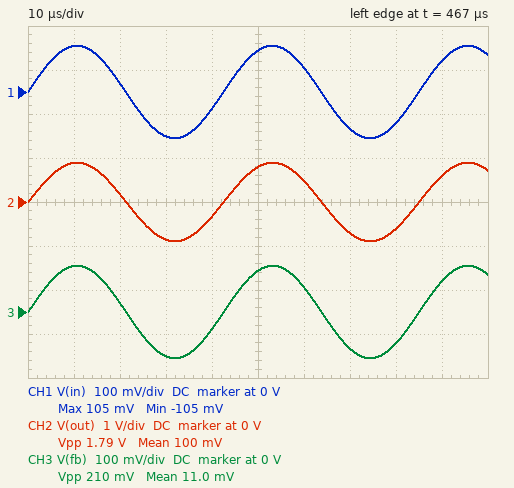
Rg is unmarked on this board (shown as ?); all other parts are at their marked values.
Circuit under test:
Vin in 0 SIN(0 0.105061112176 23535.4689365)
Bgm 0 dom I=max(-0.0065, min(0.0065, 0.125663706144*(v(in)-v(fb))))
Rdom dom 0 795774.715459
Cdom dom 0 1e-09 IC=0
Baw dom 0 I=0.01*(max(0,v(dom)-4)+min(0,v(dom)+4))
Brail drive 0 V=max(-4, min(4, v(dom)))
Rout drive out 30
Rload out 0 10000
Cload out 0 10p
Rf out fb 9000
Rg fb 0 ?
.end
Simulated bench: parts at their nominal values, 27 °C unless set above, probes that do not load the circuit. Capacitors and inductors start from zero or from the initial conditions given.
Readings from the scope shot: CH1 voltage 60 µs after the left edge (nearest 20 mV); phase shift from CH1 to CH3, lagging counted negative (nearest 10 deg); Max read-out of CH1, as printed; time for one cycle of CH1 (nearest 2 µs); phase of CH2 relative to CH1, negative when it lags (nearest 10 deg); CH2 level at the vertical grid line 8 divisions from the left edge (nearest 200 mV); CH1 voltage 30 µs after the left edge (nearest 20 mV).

60 mV
0 deg
105 mV
42 µs
0 deg
-600 mV
-100 mV
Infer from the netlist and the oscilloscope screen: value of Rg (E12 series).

1.2 kΩ
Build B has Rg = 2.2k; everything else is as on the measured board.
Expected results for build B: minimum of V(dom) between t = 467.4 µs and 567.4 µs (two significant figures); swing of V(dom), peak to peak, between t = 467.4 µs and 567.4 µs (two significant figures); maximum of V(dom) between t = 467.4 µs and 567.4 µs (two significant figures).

-540 mV
1.1 V
540 mV
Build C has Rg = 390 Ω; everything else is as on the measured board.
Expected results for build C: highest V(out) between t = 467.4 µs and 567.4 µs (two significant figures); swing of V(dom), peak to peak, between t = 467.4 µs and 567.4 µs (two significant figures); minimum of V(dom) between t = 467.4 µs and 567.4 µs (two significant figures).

2.5 V
5.1 V
-2.5 V
